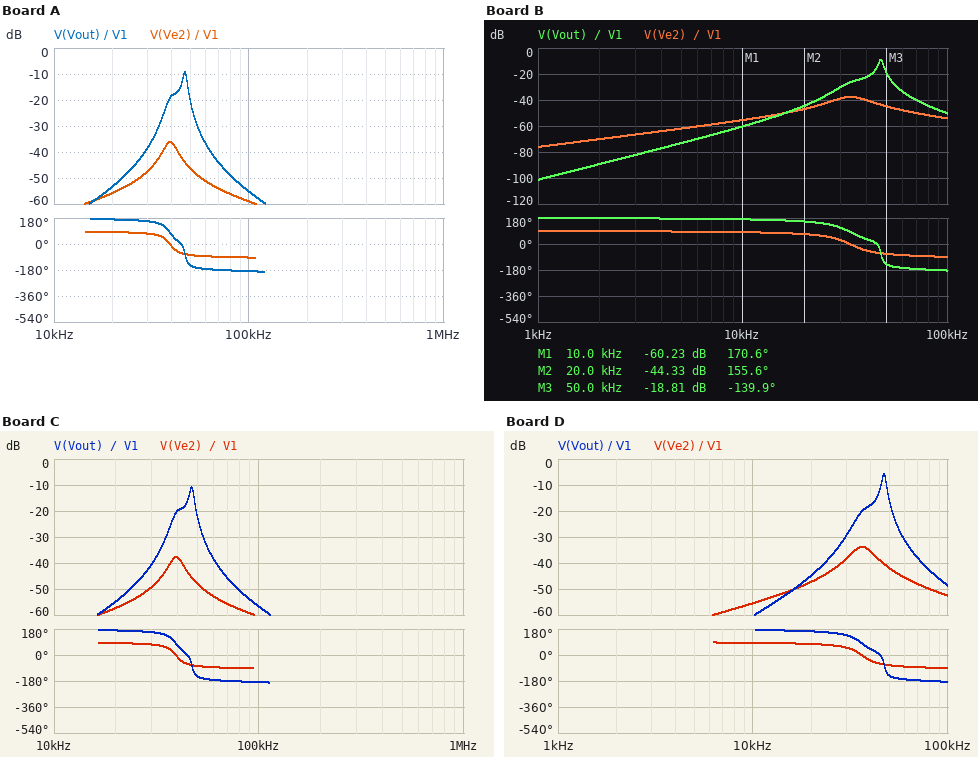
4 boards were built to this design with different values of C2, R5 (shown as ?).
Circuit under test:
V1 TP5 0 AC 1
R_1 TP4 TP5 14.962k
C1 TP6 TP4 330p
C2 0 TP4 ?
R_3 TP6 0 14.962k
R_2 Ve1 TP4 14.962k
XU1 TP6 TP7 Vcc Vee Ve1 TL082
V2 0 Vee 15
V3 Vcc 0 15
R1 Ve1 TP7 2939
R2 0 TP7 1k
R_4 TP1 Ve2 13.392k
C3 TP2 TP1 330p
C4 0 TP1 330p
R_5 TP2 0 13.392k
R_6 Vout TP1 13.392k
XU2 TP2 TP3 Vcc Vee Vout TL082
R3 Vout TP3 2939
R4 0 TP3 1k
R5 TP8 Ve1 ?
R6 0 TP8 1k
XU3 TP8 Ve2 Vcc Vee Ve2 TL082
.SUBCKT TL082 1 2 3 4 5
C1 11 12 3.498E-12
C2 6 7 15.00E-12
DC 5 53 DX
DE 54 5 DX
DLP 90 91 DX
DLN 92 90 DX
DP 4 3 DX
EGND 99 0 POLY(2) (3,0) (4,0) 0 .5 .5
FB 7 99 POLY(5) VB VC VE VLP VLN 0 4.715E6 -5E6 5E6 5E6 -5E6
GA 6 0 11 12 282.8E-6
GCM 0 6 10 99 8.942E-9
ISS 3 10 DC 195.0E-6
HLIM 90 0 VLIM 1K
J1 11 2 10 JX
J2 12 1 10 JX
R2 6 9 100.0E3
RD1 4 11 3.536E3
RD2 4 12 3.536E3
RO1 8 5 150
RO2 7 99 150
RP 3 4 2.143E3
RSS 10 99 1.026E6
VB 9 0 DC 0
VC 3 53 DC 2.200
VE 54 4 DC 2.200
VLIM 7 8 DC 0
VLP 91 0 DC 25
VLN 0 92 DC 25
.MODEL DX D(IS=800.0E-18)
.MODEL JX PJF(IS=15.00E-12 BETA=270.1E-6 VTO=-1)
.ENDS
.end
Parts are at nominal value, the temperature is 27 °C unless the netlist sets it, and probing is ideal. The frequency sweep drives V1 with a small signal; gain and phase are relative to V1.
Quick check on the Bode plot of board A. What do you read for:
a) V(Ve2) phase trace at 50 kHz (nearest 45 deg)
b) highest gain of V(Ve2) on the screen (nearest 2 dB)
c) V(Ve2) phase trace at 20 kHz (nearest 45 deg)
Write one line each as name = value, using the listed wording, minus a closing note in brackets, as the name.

V(Ve2) phase trace at 50 kHz = -90 deg
highest gain of V(Ve2) on the screen = -36 dB
V(Ve2) phase trace at 20 kHz = 90 deg
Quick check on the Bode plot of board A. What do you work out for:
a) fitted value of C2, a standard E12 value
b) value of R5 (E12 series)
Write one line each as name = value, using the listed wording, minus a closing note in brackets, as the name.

fitted value of C2, a standard E12 value = 390 pF
value of R5 = 1 MΩ
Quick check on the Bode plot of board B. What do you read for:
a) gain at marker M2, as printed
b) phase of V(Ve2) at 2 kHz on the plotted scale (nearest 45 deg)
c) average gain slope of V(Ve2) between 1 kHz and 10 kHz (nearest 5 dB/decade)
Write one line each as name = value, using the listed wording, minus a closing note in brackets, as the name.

gain at marker M2, as printed = -44.33 dB
phase of V(Ve2) at 2 kHz on the plotted scale = 90 deg
average gain slope of V(Ve2) between 1 kHz and 10 kHz = 20 dB/decade
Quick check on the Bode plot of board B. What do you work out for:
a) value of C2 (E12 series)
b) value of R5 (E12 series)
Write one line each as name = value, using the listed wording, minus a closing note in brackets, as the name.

value of C2 = 560 pF
value of R5 = 390 kΩ
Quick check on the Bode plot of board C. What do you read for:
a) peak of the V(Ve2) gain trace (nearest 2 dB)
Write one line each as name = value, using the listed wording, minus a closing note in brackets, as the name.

peak of the V(Ve2) gain trace = -38 dB
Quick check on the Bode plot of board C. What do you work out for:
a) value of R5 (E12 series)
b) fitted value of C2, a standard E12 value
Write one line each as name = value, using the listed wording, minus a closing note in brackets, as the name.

value of R5 = 1.2 MΩ
fitted value of C2, a standard E12 value = 390 pF
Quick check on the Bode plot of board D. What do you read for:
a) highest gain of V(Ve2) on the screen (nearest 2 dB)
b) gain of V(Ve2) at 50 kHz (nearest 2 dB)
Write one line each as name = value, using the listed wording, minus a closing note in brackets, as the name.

highest gain of V(Ve2) on the screen = -34 dB
gain of V(Ve2) at 50 kHz = -42 dB
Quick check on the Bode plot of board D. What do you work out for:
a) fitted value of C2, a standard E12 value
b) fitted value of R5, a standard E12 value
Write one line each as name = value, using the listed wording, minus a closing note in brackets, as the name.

fitted value of C2, a standard E12 value = 470 pF
fitted value of R5, a standard E12 value = 390 kΩ
